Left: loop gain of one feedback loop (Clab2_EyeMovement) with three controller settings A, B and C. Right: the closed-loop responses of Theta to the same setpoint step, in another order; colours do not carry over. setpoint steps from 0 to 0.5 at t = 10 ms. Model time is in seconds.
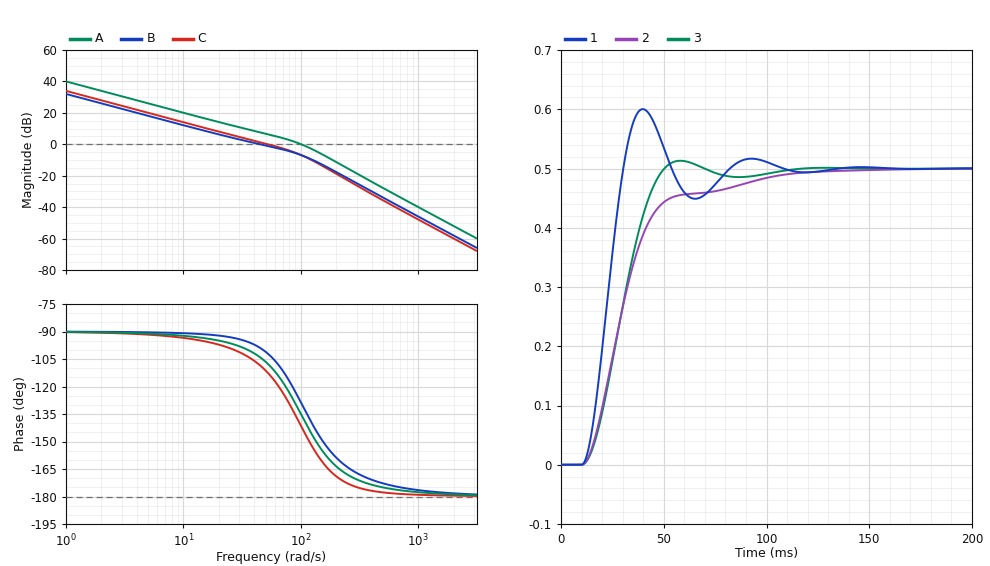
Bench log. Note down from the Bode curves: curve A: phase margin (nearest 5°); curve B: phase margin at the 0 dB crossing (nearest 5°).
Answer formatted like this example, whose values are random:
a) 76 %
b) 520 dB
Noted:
a) 45°
b) 80°
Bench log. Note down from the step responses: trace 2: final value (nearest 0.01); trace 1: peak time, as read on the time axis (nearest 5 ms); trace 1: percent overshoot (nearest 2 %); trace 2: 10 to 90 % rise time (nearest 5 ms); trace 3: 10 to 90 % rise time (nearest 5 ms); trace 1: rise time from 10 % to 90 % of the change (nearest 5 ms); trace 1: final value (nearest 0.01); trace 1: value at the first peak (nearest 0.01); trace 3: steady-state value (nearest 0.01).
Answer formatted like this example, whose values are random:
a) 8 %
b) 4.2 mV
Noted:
a) 0.50
b) 40 ms
c) 20 %
d) 35 ms
e) 25 ms
f) 15 ms
g) 0.50
h) 0.60
i) 0.50
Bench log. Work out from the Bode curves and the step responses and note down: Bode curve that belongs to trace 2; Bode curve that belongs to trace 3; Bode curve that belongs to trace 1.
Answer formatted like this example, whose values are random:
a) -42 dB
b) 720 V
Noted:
a) B
b) C
c) A
